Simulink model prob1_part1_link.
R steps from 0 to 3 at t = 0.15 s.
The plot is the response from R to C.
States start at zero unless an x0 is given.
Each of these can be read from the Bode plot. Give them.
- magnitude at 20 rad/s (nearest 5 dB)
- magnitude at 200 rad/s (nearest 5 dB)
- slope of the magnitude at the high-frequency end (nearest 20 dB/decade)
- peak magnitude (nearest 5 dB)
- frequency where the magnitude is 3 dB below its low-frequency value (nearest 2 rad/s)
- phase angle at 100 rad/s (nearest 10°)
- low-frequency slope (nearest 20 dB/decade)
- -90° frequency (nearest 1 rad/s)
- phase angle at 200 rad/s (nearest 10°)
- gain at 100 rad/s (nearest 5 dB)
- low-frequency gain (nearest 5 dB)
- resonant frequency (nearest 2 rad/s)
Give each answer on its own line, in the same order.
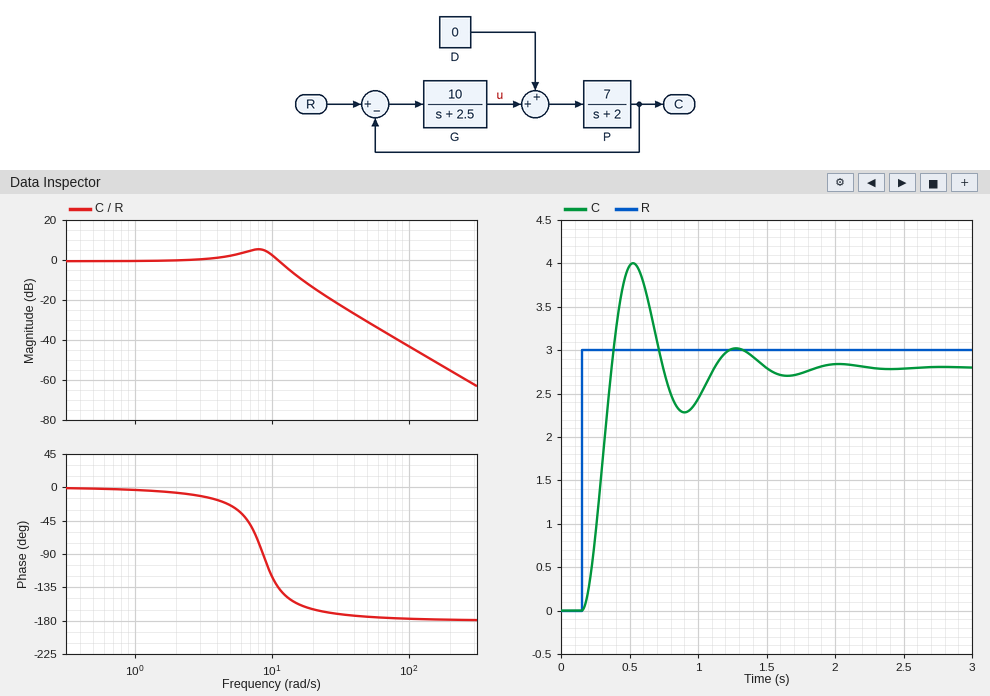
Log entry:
-15 dB
-55 dB
-40 dB/decade
5 dB
12 rad/s
-180°
0 dB/decade
9 rad/s
-180°
-45 dB
0 dB
8 rad/s
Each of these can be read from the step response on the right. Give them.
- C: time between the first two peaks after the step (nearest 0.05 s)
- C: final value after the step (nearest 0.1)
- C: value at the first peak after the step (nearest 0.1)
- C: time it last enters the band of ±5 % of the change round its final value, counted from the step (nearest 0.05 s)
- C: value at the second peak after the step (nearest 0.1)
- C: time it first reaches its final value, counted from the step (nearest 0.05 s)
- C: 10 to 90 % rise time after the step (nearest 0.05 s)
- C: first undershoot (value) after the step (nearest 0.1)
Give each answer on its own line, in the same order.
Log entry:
0.75 s
2.8
4.0
1.25 s
3.0
0.20 s
0.15 s
2.3
